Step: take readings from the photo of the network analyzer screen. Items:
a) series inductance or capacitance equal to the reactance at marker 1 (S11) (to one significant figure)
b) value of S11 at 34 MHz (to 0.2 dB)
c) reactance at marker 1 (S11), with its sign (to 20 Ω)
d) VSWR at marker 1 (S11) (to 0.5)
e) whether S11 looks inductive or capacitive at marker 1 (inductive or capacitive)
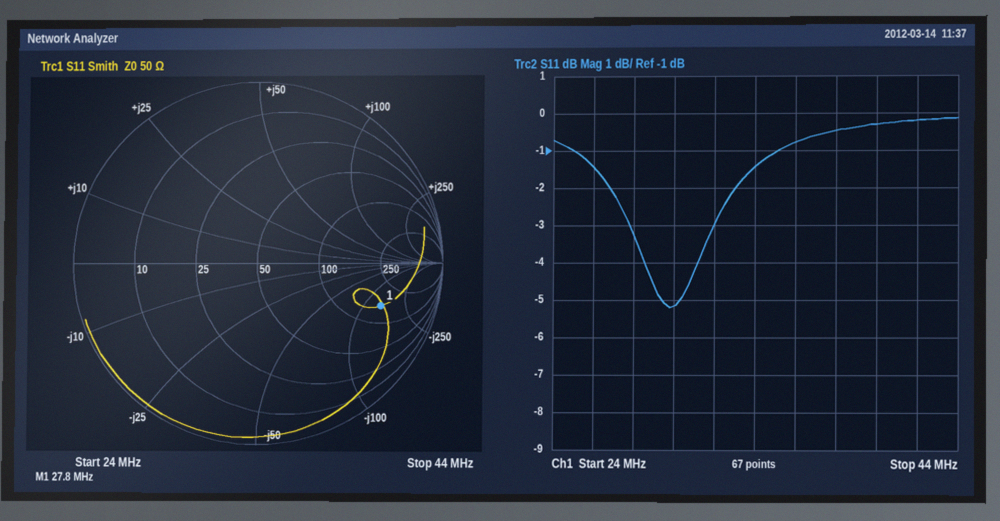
40 pF
-1.4 dB
-140 Ω
6.0
capacitive
